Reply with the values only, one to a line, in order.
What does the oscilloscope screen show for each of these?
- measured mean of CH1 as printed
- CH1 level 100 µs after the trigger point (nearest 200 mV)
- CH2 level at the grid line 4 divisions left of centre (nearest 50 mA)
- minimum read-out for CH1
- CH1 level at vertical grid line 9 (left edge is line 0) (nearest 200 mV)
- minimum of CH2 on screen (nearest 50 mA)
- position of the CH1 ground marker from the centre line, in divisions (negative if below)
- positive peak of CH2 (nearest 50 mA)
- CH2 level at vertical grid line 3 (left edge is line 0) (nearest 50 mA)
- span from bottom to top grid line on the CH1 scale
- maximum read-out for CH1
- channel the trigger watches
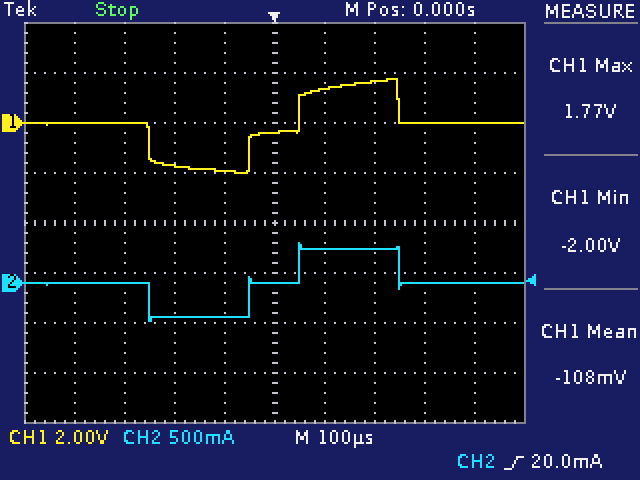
-108 mV
1.4 V
0 mA
-2.00 V
0.0 V
-400 mA
+2.0 div
400 mA
-350 mA
16 V
1.77 V
CH2
